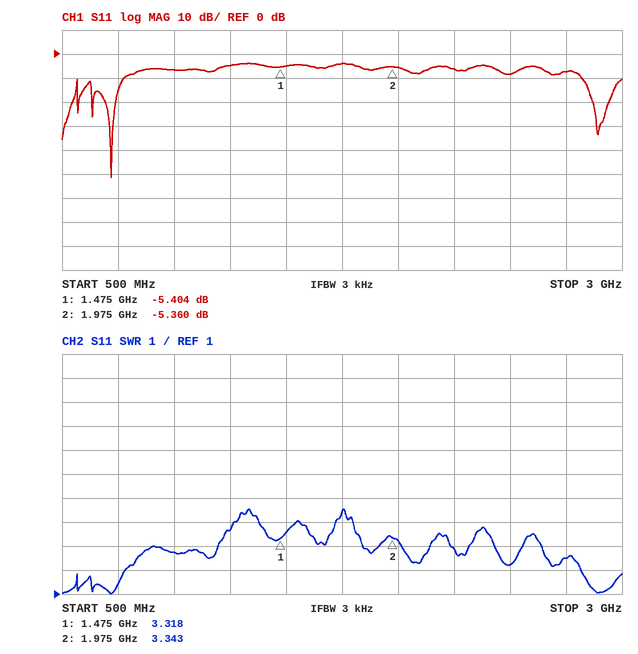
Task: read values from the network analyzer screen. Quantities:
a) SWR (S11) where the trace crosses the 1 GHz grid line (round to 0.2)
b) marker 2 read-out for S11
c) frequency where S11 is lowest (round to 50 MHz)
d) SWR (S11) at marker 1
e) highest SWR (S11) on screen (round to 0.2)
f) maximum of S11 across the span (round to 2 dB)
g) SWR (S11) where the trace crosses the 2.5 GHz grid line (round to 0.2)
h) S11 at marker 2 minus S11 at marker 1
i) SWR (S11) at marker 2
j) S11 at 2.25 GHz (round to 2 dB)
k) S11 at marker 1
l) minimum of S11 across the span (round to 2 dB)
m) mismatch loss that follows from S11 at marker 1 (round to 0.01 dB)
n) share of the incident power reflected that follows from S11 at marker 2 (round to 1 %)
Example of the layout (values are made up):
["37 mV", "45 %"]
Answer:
["2.8", "-5.360 dB", "700 MHz", "3.318", "4.6", "-4 dB", "2.2", "0.044 dB", "3.343", "-6 dB", "-5.404 dB", "-52 dB", "1.48 dB", "29 %"]
